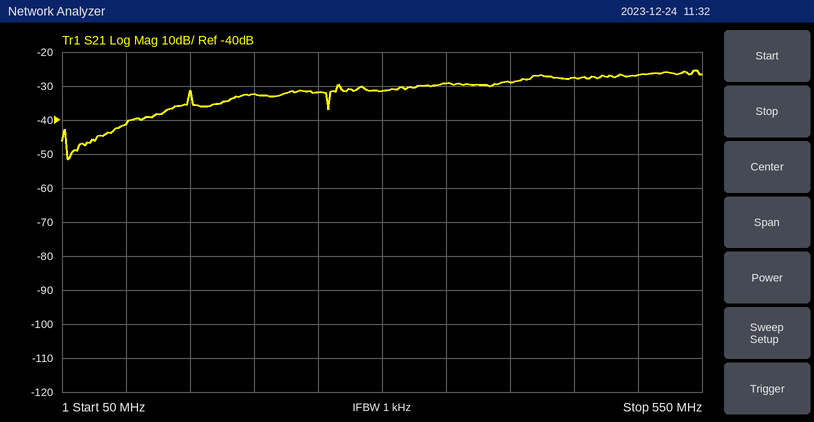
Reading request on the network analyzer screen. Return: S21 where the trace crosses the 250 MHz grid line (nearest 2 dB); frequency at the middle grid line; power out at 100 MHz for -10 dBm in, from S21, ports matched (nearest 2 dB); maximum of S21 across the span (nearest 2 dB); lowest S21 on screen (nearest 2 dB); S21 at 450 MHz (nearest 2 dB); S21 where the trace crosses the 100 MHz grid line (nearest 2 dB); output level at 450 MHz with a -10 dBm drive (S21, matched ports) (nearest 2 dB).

-32 dB
300 MHz
-52 dBm
-26 dB
-52 dB
-28 dB
-42 dB
-38 dBm
